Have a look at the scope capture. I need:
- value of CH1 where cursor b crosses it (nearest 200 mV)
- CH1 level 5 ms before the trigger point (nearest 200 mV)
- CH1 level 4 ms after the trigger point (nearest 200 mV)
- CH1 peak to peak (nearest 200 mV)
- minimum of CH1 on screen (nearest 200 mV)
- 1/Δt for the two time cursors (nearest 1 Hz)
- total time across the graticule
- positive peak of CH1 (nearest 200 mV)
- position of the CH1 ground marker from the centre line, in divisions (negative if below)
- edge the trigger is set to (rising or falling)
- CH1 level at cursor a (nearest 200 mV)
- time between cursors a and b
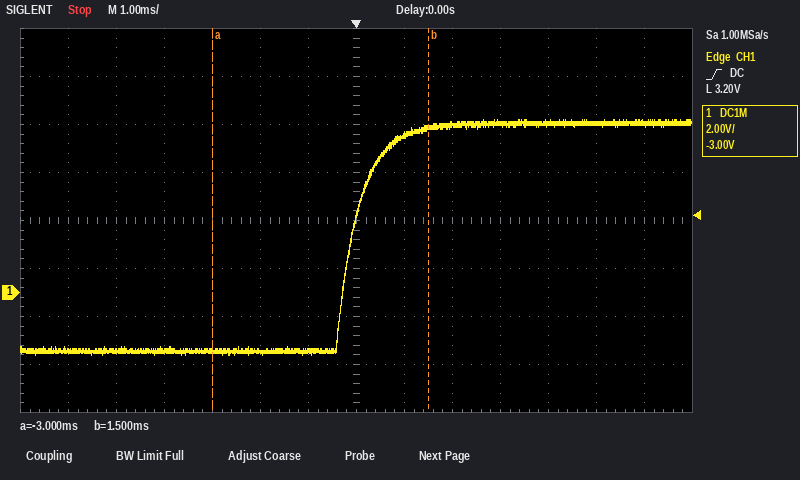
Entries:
6.8 V
-2.4 V
7.0 V
9.8 V
-2.6 V
222 Hz
14 ms
7.2 V
-1.5 div
rising
-2.4 V
4.5 ms
